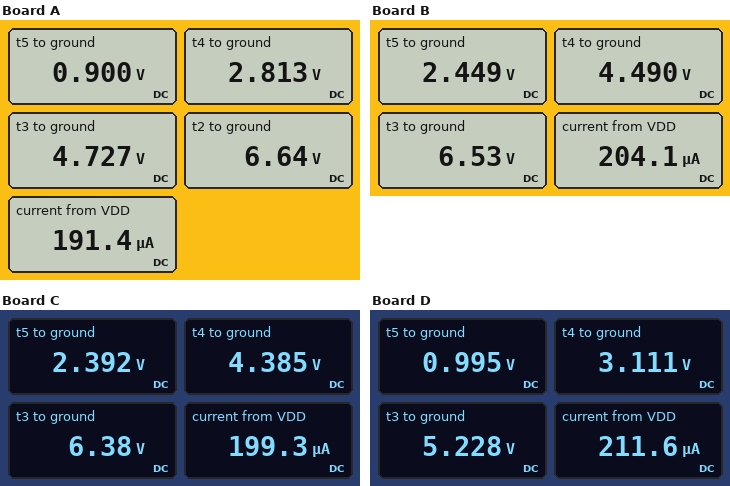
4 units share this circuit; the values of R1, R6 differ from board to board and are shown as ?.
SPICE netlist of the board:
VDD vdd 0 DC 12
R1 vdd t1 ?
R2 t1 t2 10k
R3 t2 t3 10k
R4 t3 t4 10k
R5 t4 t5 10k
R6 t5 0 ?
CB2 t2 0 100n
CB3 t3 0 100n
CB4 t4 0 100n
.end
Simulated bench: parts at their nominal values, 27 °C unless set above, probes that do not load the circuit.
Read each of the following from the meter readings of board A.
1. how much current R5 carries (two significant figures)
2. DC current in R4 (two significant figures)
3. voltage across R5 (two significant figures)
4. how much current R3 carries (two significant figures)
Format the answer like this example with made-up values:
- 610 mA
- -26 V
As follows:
- 190 µA
- 190 µA
- 1.9 V
- 190 µA
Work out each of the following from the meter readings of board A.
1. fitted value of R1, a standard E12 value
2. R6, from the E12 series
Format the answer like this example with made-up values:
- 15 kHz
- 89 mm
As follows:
- 18 kΩ
- 4.7 kΩ
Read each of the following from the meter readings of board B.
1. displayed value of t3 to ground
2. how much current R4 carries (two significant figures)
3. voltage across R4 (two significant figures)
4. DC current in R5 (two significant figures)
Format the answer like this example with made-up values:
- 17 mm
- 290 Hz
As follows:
- 6.53 V
- 200 µA
- 2.0 V
- 200 µA
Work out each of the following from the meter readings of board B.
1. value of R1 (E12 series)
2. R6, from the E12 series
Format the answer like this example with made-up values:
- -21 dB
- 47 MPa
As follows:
- 6.8 kΩ
- 12 kΩ
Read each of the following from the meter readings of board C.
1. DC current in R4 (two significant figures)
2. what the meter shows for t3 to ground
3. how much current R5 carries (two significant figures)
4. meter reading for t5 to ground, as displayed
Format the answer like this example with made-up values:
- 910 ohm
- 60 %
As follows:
- 200 µA
- 6.38 V
- 200 µA
- 2.392 V
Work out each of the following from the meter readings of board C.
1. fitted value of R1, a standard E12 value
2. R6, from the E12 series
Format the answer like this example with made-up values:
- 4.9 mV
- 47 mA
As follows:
- 8.2 kΩ
- 12 kΩ
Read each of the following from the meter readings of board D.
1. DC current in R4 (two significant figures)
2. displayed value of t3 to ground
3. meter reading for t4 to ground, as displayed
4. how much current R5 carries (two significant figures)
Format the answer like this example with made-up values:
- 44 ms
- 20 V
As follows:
- 210 µA
- 5.228 V
- 3.111 V
- 210 µA
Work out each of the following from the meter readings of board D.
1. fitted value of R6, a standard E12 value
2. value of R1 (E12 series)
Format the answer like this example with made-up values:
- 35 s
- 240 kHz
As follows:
- 4.7 kΩ
- 12 kΩ
